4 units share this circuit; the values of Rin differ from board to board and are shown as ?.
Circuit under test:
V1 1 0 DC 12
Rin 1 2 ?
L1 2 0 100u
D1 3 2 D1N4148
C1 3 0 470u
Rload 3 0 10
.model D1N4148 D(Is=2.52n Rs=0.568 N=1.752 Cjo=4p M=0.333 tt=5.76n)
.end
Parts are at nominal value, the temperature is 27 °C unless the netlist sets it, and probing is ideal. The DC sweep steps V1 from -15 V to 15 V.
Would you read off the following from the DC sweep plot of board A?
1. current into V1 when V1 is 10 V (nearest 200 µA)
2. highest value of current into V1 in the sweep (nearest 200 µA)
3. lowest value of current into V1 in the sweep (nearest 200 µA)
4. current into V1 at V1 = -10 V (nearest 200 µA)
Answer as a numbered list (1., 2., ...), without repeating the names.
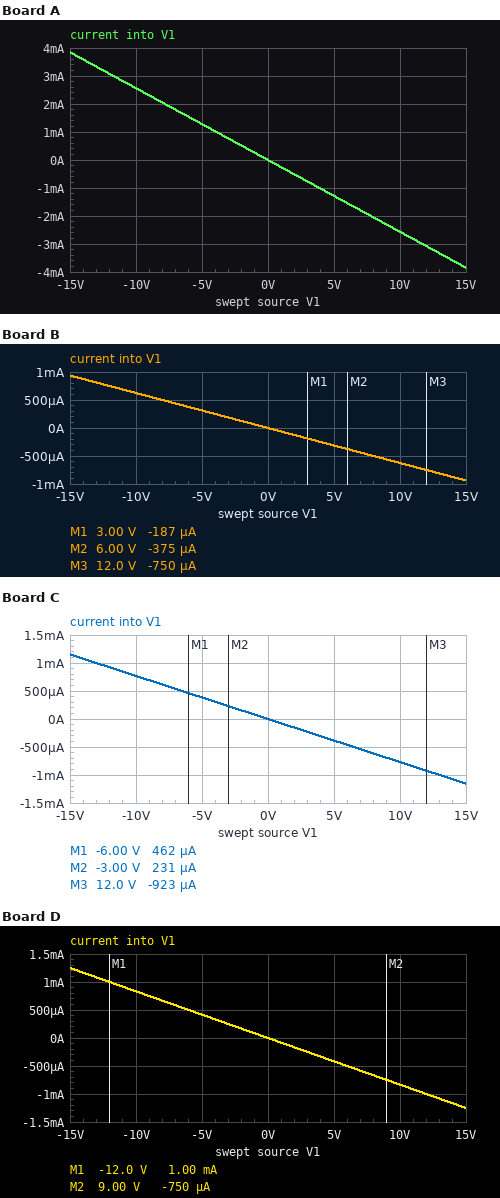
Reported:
1. -2.6 mA
2. 3.8 mA
3. -3.8 mA
4. 2.6 mA
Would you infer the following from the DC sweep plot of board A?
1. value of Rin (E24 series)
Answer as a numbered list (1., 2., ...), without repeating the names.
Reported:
1. 3.9 kΩ
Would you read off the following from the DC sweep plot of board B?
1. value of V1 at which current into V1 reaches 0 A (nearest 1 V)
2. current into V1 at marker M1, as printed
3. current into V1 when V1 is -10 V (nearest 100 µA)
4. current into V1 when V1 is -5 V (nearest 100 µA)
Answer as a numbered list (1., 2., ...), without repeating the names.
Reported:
1. 0 V
2. -187 µA
3. 600 µA
4. 300 µA
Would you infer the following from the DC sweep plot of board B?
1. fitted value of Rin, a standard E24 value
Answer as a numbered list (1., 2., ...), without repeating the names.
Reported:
1. 16 kΩ
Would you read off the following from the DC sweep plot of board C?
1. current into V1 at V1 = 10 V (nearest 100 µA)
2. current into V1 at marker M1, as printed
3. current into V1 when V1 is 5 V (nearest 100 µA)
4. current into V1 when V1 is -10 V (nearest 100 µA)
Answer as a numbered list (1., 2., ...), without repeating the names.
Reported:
1. -800 µA
2. 462 µA
3. -400 µA
4. 800 µA
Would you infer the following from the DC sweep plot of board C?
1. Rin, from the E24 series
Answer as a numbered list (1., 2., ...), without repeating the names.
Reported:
1. 13 kΩ
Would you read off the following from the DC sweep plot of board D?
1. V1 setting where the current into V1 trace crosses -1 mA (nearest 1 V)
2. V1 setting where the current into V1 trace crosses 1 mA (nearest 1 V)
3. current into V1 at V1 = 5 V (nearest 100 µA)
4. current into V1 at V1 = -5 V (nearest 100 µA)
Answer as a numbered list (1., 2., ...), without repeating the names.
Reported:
1. 12 V
2. -12 V
3. -400 µA
4. 400 µA
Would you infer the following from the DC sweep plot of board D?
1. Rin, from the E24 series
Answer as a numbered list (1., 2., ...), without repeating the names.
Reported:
1. 12 kΩ
